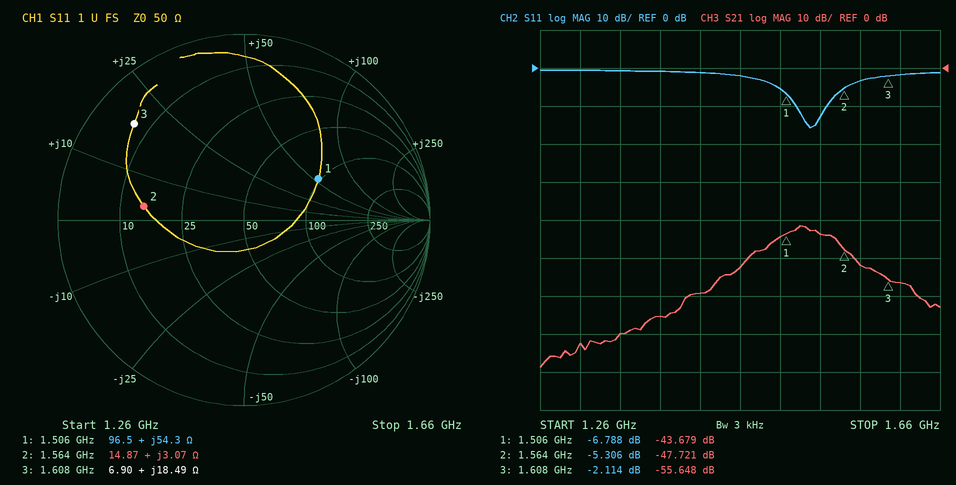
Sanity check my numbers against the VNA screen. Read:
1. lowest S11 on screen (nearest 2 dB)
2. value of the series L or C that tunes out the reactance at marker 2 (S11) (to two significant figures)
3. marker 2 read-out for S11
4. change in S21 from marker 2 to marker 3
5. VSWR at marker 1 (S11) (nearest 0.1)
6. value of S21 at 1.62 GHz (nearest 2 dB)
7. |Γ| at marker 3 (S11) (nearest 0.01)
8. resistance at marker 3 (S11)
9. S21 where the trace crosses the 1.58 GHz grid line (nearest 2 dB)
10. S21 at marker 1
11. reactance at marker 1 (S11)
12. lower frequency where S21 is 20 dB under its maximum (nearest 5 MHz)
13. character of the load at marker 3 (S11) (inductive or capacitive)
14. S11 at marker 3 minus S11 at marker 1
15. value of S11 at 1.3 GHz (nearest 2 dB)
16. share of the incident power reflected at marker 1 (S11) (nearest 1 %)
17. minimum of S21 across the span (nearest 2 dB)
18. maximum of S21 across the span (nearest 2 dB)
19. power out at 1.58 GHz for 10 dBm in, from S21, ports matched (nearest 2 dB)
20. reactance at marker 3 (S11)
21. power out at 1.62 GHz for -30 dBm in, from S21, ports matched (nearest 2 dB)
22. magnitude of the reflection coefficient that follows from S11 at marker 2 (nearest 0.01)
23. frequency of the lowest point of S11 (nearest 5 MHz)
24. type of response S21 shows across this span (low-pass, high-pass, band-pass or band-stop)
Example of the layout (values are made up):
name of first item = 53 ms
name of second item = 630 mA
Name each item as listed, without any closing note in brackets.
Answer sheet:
lowest S11 on screen = -16 dB
value of the series L or C that tunes out the reactance at marker 2 (S11) = 33 pF
marker 2 read-out for S11 = -5.306 dB
change in S21 from marker 2 to marker 3 = -7.927 dB
VSWR at marker 1 (S11) = 2.7
value of S21 at 1.62 GHz = -56 dB
|Γ| at marker 3 (S11) = 0.78
resistance at marker 3 = 6.90 Ω
S21 where the trace crosses the 1.58 GHz grid line = -52 dB
S21 at marker 1 = -43.679 dB
reactance at marker 1 = +54.3 Ω
lower frequency where S21 is 20 dB under its maximum = 1.405 GHz
character of the load at marker 3 (S11) = inductive
S11 at marker 3 minus S11 at marker 1 = 4.674 dB
value of S11 at 1.3 GHz = 0 dB
share of the incident power reflected at marker 1 (S11) = 21 %
minimum of S21 across the span = -78 dB
maximum of S21 across the span = -42 dB
power out at 1.58 GHz for 10 dBm in, from S21, ports matched = -42 dBm
reactance at marker 3 = +18.49 Ω
power out at 1.62 GHz for -30 dBm in, from S21, ports matched = -86 dBm
magnitude of the reflection coefficient that follows from S11 at marker 2 = 0.54
frequency of the lowest point of S11 = 1.530 GHz
type of response S21 shows across this span = band-pass
